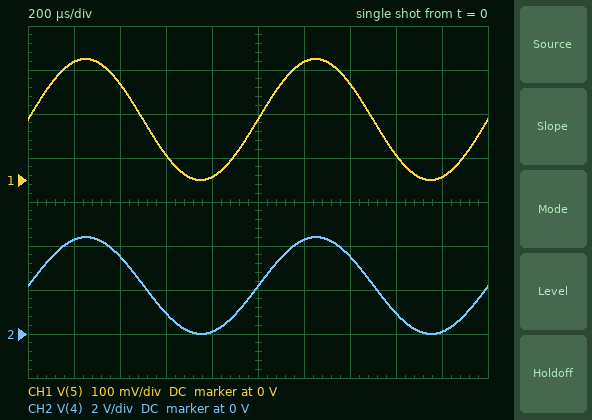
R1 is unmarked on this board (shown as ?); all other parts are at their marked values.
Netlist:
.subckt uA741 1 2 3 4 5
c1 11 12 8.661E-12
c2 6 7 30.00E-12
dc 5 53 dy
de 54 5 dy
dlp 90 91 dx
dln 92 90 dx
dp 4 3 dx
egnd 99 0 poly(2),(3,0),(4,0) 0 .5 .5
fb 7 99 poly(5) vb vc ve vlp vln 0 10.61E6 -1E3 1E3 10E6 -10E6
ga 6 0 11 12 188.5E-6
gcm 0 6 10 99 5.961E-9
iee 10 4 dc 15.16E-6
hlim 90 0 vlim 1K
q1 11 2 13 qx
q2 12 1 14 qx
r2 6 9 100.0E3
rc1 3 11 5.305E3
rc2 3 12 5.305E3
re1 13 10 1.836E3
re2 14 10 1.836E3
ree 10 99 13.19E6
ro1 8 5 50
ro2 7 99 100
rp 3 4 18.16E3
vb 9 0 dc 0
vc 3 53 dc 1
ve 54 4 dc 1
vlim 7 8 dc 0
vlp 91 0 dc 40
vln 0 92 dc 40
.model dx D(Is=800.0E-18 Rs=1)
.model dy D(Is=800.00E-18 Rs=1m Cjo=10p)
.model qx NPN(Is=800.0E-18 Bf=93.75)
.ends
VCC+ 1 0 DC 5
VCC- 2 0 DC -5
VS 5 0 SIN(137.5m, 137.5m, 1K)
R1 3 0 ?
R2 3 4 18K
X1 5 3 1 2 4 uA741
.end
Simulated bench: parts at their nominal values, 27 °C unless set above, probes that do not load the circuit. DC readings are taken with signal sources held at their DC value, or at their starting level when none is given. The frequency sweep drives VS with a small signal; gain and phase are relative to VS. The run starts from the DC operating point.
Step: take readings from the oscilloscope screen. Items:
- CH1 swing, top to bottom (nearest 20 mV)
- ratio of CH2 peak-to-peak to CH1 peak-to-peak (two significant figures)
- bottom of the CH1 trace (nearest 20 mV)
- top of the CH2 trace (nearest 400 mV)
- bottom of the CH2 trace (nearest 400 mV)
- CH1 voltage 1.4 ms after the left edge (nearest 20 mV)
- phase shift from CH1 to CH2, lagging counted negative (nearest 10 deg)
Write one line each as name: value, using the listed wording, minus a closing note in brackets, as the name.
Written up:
CH1 swing, top to bottom: 280 mV
ratio of CH2 peak-to-peak to CH1 peak-to-peak: 16
bottom of the CH1 trace: 0 V
top of the CH2 trace: 4.4 V
bottom of the CH2 trace: 0 V
CH1 voltage 1.4 ms after the left edge: 220 mV
phase shift from CH1 to CH2, lagging counted negative: 0 deg
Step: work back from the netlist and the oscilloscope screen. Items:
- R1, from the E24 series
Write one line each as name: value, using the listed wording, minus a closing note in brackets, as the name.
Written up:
R1, from the E24 series: 1.2 kΩ
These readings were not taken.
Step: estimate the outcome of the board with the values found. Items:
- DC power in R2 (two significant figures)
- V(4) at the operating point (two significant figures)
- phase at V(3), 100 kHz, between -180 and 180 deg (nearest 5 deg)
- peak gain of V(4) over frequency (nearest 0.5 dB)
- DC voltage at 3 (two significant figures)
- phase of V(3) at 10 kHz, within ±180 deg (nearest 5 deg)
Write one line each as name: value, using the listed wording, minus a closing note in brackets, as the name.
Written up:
DC power in R2: 240 µW
V(4) at the operating point: 2.2 V
phase at V(3), 100 kHz, between -180 and 180 deg: -60 deg
peak gain of V(4) over frequency: 24.0 dB
DC voltage at 3: 140 mV
phase of V(3) at 10 kHz, within ±180 deg: -10 deg
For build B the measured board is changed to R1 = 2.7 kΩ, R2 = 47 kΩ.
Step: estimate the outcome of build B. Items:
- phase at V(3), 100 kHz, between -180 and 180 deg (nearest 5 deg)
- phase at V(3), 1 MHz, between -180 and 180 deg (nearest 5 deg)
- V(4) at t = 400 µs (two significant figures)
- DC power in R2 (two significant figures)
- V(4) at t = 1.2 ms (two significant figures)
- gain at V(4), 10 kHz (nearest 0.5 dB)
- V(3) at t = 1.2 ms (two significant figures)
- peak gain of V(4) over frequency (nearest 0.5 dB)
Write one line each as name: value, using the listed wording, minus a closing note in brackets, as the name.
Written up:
phase at V(3), 100 kHz, between -180 and 180 deg: -65 deg
phase at V(3), 1 MHz, between -180 and 180 deg: -115 deg
V(4) at t = 400 µs: 4.1 V
DC power in R2: 120 µW
V(4) at t = 1.2 ms: 4.8 V
gain at V(4), 10 kHz: 25.0 dB
V(3) at t = 1.2 ms: 260 mV
peak gain of V(4) over frequency: 25.5 dB
